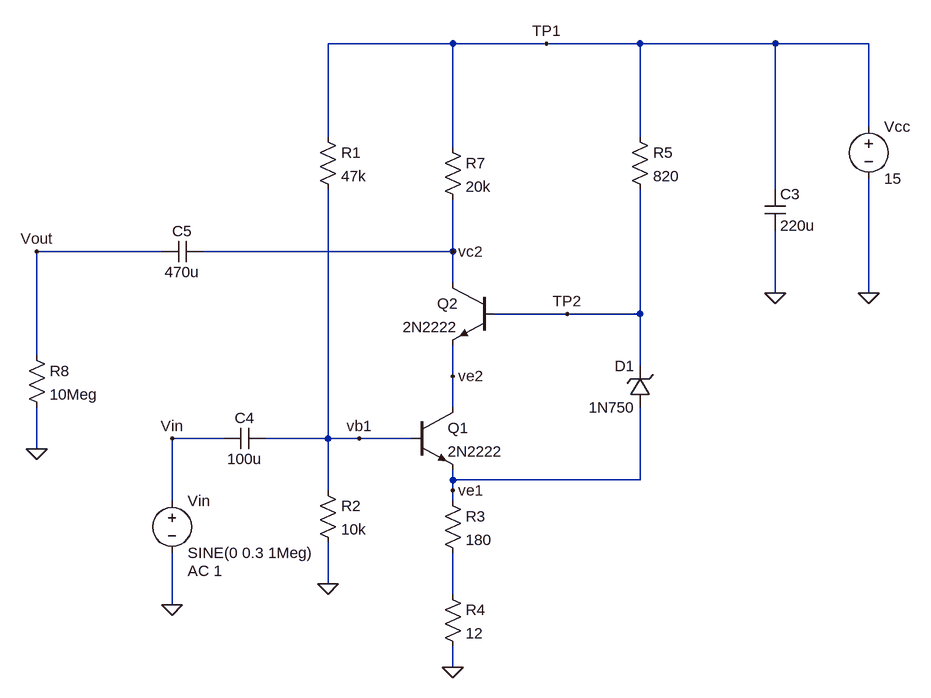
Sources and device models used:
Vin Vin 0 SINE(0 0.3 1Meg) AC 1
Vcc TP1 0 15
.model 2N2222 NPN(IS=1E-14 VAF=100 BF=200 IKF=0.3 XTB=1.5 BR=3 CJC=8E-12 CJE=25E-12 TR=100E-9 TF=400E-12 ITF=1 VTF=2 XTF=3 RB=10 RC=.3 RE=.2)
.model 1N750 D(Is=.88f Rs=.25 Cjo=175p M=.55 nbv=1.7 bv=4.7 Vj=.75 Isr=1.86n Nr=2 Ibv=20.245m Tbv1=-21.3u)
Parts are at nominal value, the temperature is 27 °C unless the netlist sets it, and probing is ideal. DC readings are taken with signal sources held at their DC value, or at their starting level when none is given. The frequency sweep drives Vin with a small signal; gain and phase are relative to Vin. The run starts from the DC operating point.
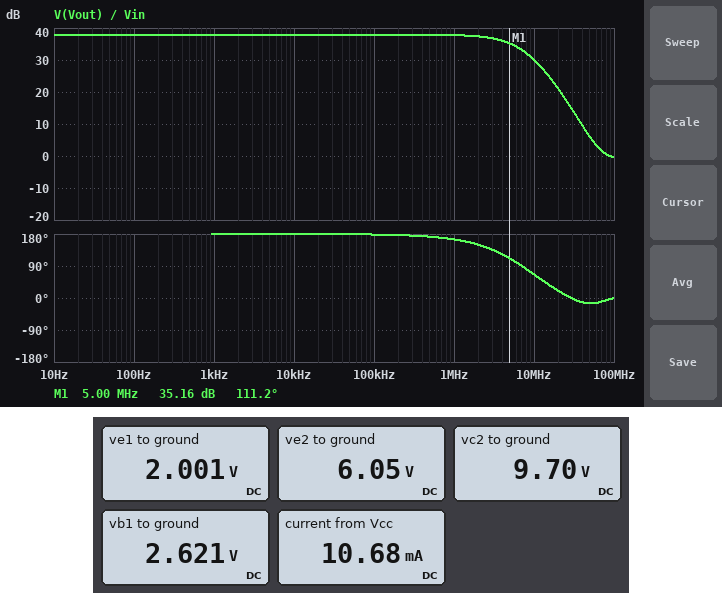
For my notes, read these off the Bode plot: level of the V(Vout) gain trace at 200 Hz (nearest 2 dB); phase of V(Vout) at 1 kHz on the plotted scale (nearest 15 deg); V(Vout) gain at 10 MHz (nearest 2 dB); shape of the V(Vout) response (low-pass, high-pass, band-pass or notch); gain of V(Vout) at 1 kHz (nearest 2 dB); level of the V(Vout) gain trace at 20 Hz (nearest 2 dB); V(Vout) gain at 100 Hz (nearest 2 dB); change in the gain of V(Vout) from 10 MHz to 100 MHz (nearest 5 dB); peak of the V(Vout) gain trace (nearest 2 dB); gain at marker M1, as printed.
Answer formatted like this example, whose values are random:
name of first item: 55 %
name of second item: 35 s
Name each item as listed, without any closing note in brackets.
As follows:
level of the V(Vout) gain trace at 200 Hz: 38 dB
phase of V(Vout) at 1 kHz on the plotted scale: 180 deg
V(Vout) gain at 10 MHz: 30 dB
shape of the V(Vout) response: low-pass
gain of V(Vout) at 1 kHz: 38 dB
level of the V(Vout) gain trace at 20 Hz: 38 dB
V(Vout) gain at 100 Hz: 38 dB
change in the gain of V(Vout) from 10 MHz to 100 MHz: -30 dB
peak of the V(Vout) gain trace: 38 dB
gain at marker M1, as printed: 35.16 dB
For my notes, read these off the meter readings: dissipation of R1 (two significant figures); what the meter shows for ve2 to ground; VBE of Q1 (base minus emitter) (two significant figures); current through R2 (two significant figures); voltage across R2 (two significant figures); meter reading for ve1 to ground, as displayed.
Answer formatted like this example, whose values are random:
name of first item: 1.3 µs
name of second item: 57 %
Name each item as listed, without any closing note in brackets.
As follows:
dissipation of R1: 3.3 mW
what the meter shows for ve2 to ground: 6.05 V
VBE of Q1 (base minus emitter): 620 mV
current through R2: 260 µA
voltage across R2: 2.6 V
meter reading for ve1 to ground, as displayed: 2.001 V
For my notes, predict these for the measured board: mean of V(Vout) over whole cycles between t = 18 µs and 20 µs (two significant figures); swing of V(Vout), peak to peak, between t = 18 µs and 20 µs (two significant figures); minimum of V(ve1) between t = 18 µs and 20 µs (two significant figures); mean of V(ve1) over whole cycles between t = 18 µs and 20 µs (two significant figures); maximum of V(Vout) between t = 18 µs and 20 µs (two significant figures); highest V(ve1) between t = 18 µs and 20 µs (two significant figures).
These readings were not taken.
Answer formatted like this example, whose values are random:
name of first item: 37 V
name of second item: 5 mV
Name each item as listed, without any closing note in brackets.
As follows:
mean of V(Vout) over whole cycles between t = 18 µs and 20 µs: -3.9 V
swing of V(Vout), peak to peak, between t = 18 µs and 20 µs: 820 mV
minimum of V(ve1) between t = 18 µs and 20 µs: 2.0 V
mean of V(ve1) over whole cycles between t = 18 µs and 20 µs: 2.1 V
maximum of V(Vout) between t = 18 µs and 20 µs: -3.7 V
highest V(ve1) between t = 18 µs and 20 µs: 2.2 V
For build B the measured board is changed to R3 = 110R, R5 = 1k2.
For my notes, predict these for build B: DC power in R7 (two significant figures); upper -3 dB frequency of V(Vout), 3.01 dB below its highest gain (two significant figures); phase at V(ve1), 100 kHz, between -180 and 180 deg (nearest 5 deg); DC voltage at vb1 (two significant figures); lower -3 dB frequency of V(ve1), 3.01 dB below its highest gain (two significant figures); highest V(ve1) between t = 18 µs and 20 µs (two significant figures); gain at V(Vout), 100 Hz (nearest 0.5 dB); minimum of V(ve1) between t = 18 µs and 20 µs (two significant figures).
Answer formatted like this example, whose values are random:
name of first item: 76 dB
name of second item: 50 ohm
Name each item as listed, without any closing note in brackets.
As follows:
DC power in R7: 9.0 mW
upper -3 dB frequency of V(Vout), 3.01 dB below its highest gain: 1.9 MHz
phase at V(ve1), 100 kHz, between -180 and 180 deg: 0 deg
DC voltage at vb1: 2.1 V
lower -3 dB frequency of V(ve1), 3.01 dB below its highest gain: 3.5 Hz
highest V(ve1) between t = 18 µs and 20 µs: 1.6 V
gain at V(Vout), 100 Hz: 16.0 dB
minimum of V(ve1) between t = 18 µs and 20 µs: 1.1 V
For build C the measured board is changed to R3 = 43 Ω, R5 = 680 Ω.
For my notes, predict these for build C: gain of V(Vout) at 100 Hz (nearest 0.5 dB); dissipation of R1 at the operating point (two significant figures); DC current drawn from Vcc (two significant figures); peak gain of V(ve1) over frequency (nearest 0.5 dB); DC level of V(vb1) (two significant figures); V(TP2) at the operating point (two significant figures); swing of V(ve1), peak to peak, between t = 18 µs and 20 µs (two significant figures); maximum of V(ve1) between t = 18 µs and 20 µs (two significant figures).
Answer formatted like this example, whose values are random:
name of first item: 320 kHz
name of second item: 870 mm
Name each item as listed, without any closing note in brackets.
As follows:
gain of V(Vout) at 100 Hz: 21.5 dB
dissipation of R1 at the operating point: 3.7 mW
DC current drawn from Vcc: 19 mA
peak gain of V(ve1) over frequency: -0.5 dB
DC level of V(vb1): 1.8 V
V(TP2) at the operating point: 2.5 V
swing of V(ve1), peak to peak, between t = 18 µs and 20 µs: 500 mV
maximum of V(ve1) between t = 18 µs and 20 µs: 1.3 V
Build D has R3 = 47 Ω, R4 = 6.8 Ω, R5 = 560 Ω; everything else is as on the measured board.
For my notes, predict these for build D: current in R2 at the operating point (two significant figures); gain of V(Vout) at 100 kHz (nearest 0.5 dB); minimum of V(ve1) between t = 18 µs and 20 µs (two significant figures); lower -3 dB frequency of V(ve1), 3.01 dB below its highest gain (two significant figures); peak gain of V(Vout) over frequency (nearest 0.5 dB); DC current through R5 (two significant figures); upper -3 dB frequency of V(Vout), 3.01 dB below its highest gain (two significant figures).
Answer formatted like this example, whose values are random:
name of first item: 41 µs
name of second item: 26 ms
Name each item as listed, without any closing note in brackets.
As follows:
current in R2 at the operating point: 180 µA
gain of V(Vout) at 100 kHz: 20.0 dB
minimum of V(ve1) between t = 18 µs and 20 µs: 920 mV
lower -3 dB frequency of V(ve1), 3.01 dB below its highest gain: 370 mHz
peak gain of V(Vout) over frequency: 21.0 dB
DC current through R5: 19 mA
upper -3 dB frequency of V(Vout), 3.01 dB below its highest gain: 39 MHz
